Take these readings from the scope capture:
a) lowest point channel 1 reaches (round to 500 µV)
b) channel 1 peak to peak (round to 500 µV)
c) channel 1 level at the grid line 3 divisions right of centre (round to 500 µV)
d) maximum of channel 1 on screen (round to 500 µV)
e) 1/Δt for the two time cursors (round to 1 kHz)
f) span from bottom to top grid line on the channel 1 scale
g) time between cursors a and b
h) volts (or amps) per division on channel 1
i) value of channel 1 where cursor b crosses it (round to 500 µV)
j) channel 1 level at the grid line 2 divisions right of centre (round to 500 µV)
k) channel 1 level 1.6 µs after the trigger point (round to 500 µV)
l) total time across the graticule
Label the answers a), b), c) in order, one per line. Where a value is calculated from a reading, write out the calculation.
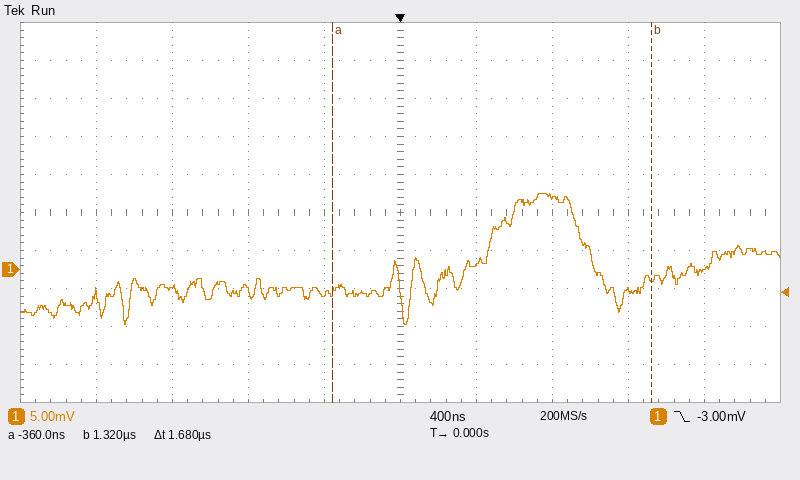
a) -7.0 mV
b) 10.0 mV − (-7.0 mV) = 17.0 mV
c) -3.0 mV
d) 10.0 mV
e) 1 / 1.68 µs ≈ 595 kHz
f) 50 mV
g) 1.68 µs
h) 5 mV
i) -1.0 mV
j) 9.5 mV
k) 0.0 mV
l) 4 µs
